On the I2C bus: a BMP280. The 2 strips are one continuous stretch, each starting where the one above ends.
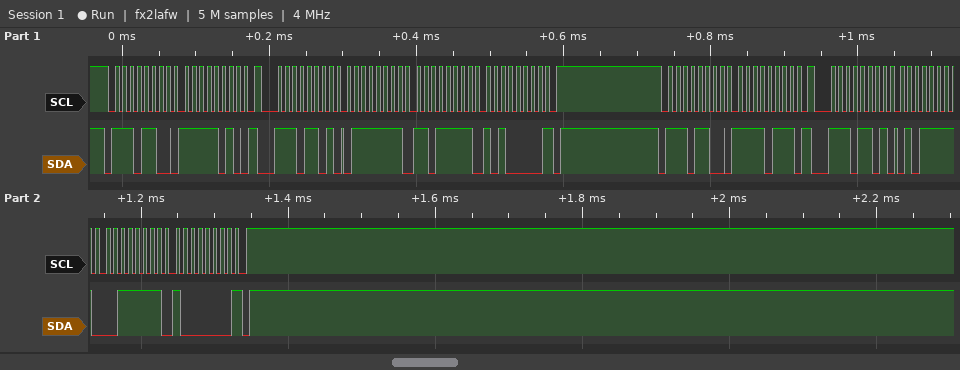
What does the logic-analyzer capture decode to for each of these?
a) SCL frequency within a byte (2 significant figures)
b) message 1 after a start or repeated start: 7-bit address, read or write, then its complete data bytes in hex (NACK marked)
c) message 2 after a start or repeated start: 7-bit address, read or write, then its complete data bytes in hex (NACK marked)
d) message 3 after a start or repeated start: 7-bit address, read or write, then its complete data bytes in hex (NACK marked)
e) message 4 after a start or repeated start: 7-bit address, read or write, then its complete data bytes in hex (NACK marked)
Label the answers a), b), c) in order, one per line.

a) 100 kHz
b) 0x76 write: FA
c) 0x76 read: 7F DF A0 NACK
d) 0x76 write: F7
e) 0x76 read: 5F 3F 80 NACK
